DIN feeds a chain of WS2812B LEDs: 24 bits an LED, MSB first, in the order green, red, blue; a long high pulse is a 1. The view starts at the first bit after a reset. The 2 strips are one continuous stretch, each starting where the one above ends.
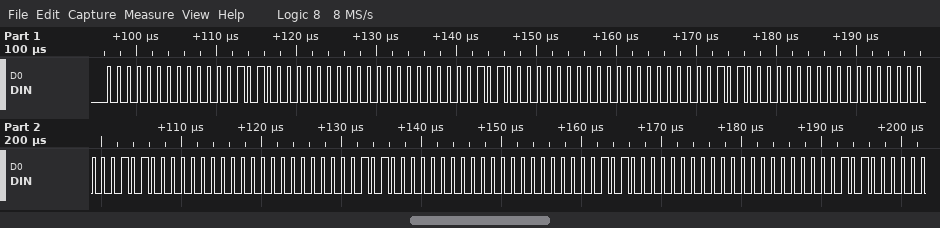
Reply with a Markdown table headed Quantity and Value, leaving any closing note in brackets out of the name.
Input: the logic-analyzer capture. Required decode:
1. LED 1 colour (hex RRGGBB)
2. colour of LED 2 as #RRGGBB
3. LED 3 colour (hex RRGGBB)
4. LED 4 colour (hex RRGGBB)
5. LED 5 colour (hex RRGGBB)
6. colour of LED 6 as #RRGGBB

| Quantity | Value |
|---|---|
| LED 1 colour | #050000 |
| colour of LED 2 as #RRGGBB | #050000 |
| LED 3 colour | #050000 |
| LED 4 colour | #050000 |
| LED 5 colour | #050000 |
| colour of LED 6 as #RRGGBB | #050000 |
